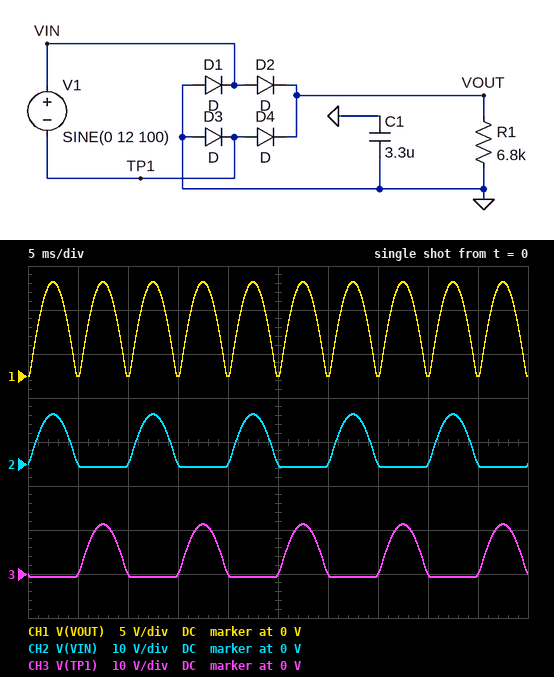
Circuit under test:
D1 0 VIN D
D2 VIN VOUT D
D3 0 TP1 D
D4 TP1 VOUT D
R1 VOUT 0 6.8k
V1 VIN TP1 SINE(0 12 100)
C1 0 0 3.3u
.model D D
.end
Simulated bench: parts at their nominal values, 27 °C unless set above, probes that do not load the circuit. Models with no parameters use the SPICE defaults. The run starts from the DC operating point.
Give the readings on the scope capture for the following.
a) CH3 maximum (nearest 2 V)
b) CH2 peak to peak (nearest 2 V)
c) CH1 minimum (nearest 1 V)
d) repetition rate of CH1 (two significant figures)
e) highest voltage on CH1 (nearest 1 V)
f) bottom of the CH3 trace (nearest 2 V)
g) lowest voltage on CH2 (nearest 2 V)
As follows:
12 V
12 V
0 V
200 Hz
11 V
0 V
0 V
